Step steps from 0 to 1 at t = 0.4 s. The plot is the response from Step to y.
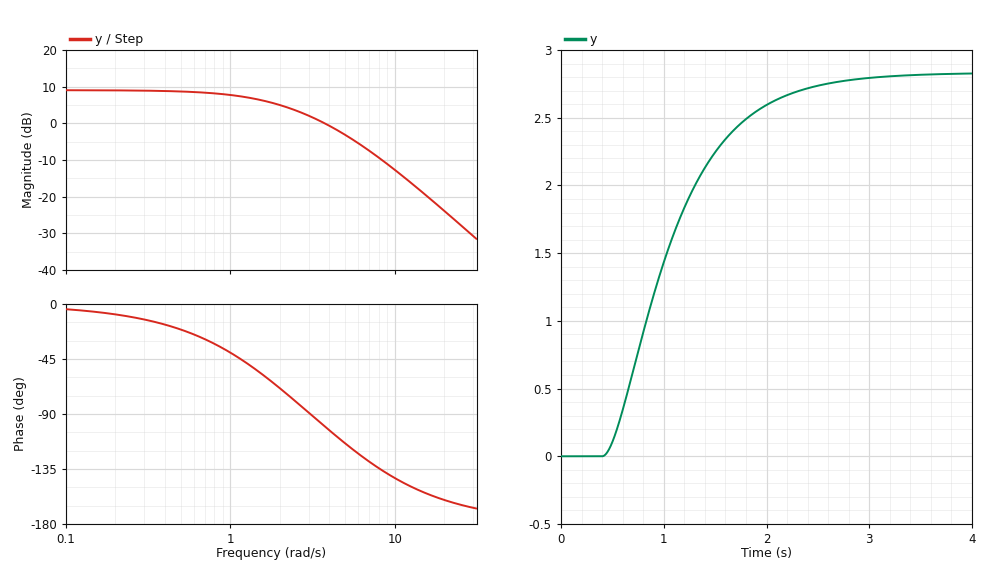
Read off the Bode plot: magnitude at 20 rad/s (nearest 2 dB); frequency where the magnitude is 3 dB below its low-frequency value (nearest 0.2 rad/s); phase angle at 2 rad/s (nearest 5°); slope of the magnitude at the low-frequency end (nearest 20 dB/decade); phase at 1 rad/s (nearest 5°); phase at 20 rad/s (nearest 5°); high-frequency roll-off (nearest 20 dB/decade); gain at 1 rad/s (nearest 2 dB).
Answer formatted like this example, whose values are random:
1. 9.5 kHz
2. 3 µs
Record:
1. -24 dB
2. 1.6 rad/s
3. -70°
4. 0 dB/decade
5. -40°
6. -160°
7. -40 dB/decade
8. 8 dB
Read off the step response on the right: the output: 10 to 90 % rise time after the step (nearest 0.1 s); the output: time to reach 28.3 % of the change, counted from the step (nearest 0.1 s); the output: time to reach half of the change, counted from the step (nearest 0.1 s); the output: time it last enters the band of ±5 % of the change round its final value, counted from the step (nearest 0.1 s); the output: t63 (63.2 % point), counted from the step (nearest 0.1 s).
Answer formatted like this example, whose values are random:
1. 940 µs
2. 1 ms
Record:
1. 1.3 s
2. 0.4 s
3. 0.6 s
4. 1.9 s
5. 0.8 s
